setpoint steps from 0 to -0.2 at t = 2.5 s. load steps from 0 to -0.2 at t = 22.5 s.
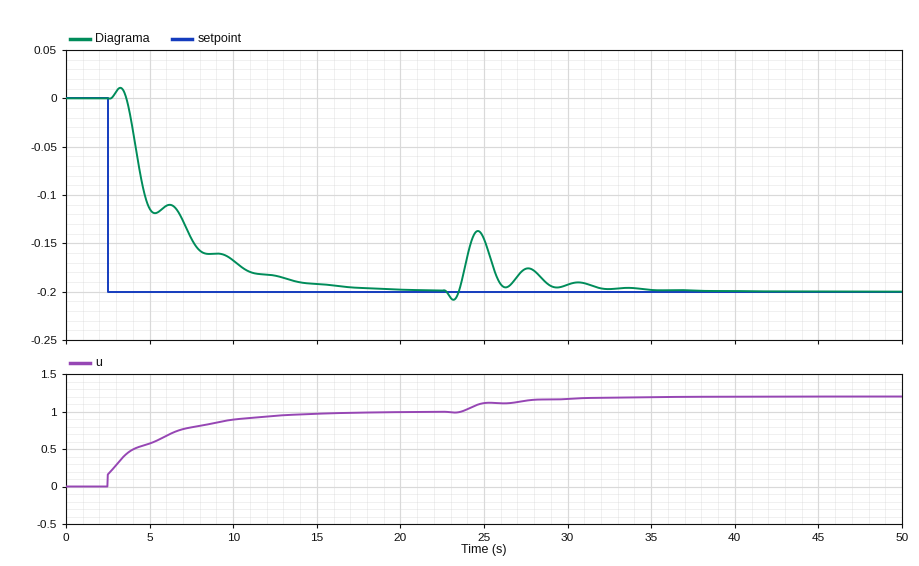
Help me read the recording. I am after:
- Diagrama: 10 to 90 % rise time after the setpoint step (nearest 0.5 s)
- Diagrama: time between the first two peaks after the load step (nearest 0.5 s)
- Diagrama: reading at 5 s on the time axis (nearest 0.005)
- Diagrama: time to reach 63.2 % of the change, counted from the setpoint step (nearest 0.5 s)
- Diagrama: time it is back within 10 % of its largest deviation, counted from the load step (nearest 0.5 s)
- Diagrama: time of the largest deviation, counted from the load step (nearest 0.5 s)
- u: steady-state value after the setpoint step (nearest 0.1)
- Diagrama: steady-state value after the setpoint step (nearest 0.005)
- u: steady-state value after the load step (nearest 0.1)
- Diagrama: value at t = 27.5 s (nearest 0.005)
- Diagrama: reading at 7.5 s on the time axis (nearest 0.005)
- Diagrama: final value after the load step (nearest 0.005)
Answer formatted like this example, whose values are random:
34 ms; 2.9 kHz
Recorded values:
7.0 s; 3.0 s; -0.115; 4.5 s; 9.0 s; 2.0 s; 1.0; -0.200; 1.2; -0.175; -0.145; -0.200
